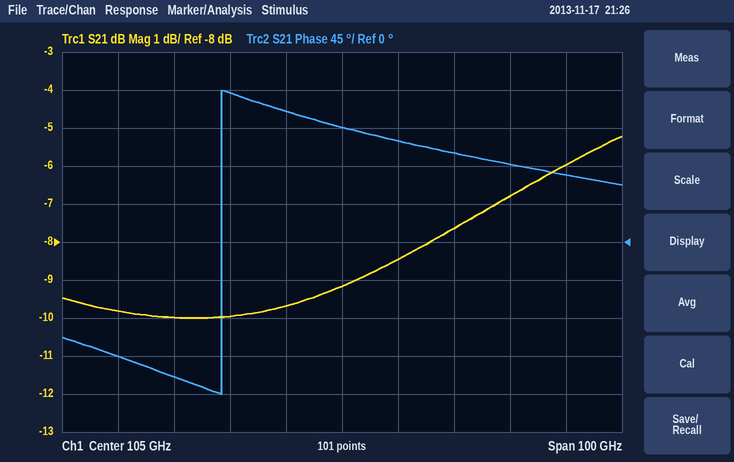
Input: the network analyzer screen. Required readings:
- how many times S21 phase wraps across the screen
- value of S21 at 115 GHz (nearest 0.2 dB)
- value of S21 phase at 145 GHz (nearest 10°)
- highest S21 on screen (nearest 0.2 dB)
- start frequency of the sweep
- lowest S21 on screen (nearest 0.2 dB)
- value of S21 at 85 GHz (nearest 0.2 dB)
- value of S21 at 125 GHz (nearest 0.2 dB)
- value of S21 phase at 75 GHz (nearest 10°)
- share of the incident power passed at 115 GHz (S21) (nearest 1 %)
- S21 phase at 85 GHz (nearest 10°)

1
-8.4 dB
80°
-5.2 dB
55 GHz
-10.0 dB
-10.0 dB
-7.6 dB
-160°
14 %
180°
